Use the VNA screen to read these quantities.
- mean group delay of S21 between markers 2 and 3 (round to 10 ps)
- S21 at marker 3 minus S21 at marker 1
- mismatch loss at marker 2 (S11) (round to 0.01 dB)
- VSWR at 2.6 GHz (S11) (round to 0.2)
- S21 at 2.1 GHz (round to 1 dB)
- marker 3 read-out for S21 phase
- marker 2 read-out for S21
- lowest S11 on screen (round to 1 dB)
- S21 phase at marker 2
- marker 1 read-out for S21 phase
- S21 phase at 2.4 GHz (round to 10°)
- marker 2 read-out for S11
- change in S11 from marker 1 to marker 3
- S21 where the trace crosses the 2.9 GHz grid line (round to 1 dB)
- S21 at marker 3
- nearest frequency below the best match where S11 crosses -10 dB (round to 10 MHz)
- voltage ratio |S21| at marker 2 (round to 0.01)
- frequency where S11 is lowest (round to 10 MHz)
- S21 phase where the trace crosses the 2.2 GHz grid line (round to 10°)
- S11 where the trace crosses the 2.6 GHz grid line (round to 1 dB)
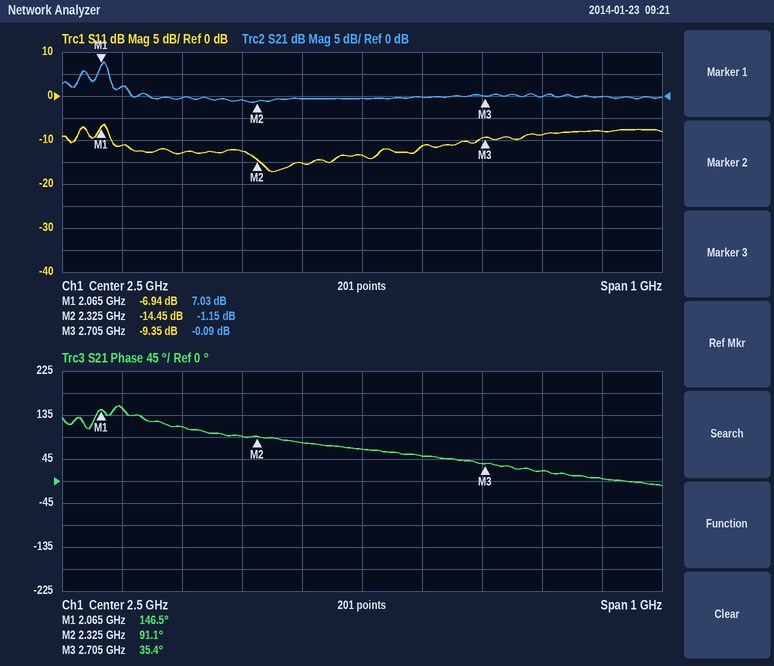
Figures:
410 ps
-7.12 dB
0.16 dB
1.8
2 dB
35.4°
-1.15 dB
-17 dB
91.1°
146.5°
80°
-14.45 dB
-2.41 dB
0 dB
-0.09 dB
2.08 GHz
0.88
2.35 GHz
110°
-11 dB
